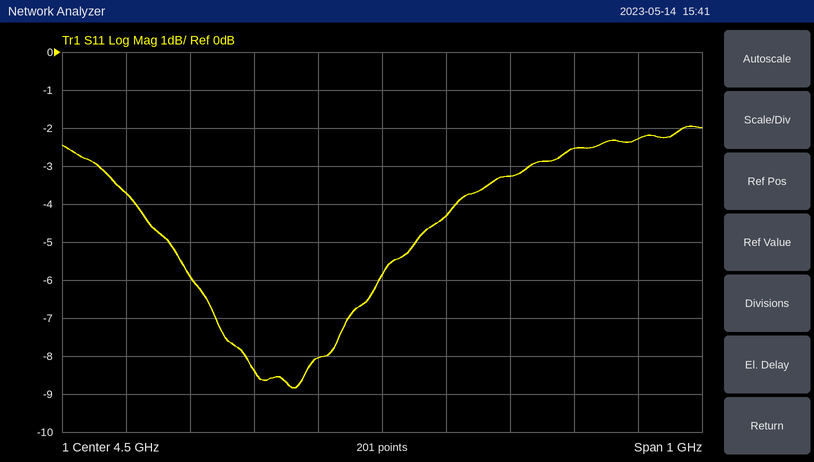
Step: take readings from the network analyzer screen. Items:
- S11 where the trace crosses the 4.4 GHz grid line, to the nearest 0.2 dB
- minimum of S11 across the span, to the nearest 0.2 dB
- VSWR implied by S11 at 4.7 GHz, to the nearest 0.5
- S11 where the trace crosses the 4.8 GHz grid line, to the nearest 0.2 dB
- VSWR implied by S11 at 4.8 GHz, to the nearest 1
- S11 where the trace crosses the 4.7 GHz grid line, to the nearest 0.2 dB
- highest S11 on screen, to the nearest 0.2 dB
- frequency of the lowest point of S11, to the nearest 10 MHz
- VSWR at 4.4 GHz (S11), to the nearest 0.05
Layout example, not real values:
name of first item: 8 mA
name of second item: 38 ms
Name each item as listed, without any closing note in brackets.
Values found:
S11 where the trace crosses the 4.4 GHz grid line, to the nearest 0.2 dB: -8.0 dB
minimum of S11 across the span, to the nearest 0.2 dB: -8.8 dB
VSWR implied by S11 at 4.7 GHz, to the nearest 0.5: 5.5
S11 where the trace crosses the 4.8 GHz grid line, to the nearest 0.2 dB: -2.6 dB
VSWR implied by S11 at 4.8 GHz, to the nearest 1: 7
S11 where the trace crosses the 4.7 GHz grid line, to the nearest 0.2 dB: -3.2 dB
highest S11 on screen, to the nearest 0.2 dB: -2.0 dB
frequency of the lowest point of S11, to the nearest 10 MHz: 4.36 GHz
VSWR at 4.4 GHz (S11), to the nearest 0.05: 2.30
